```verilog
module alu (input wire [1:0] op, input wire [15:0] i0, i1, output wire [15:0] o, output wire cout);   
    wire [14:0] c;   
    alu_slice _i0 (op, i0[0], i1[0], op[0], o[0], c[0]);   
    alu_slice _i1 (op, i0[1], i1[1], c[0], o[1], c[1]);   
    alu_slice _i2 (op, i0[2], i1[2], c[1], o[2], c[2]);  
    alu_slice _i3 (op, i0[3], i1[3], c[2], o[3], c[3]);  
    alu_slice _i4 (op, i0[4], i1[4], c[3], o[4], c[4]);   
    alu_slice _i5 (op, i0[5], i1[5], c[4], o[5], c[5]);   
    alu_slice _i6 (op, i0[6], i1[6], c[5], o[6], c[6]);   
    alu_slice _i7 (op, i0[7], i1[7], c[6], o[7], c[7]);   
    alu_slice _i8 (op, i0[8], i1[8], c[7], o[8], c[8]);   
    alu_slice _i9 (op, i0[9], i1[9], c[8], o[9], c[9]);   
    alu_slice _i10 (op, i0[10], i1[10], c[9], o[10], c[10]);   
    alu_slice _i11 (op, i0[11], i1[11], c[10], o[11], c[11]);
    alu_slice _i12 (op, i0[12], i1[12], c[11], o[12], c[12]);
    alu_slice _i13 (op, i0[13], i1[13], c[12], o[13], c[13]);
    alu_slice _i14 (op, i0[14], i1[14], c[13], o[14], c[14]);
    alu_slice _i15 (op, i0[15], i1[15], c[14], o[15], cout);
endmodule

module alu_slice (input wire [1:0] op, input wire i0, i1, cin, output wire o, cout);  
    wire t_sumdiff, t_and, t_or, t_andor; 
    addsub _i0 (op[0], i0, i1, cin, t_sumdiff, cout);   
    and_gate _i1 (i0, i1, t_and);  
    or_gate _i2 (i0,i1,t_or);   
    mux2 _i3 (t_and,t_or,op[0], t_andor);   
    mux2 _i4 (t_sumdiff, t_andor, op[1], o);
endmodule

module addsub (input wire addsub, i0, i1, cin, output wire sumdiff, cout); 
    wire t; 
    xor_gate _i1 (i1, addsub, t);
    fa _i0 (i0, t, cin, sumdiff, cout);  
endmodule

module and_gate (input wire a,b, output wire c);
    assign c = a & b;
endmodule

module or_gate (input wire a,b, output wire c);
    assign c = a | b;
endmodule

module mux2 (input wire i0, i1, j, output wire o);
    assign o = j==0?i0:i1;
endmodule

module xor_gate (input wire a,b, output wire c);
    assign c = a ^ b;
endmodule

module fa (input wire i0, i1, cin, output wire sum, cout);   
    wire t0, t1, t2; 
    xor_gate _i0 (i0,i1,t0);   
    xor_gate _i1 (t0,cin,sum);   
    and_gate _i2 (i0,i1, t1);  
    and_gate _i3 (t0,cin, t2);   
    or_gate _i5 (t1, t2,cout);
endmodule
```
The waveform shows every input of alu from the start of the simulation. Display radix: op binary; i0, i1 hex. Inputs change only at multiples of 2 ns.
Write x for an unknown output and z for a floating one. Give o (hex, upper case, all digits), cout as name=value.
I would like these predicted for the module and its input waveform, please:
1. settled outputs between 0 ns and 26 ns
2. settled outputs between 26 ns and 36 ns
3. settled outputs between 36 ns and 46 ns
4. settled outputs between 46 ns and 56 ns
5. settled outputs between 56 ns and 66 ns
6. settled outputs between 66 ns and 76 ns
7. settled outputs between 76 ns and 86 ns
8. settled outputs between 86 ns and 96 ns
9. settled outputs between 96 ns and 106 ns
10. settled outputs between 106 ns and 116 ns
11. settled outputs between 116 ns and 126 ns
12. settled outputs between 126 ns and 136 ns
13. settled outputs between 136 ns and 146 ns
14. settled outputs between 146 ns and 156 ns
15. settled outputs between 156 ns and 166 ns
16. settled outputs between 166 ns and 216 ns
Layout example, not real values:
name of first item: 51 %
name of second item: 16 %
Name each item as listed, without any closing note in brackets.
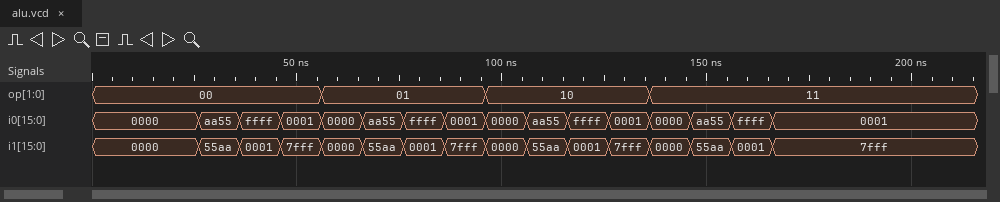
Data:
settled outputs between 0 ns and 26 ns: o=0000, cout=0
settled outputs between 26 ns and 36 ns: o=FFFF, cout=0
settled outputs between 36 ns and 46 ns: o=0000, cout=1
settled outputs between 46 ns and 56 ns: o=8000, cout=0
settled outputs between 56 ns and 66 ns: o=0000, cout=1
settled outputs between 66 ns and 76 ns: o=54AB, cout=1
settled outputs between 76 ns and 86 ns: o=FFFE, cout=1
settled outputs between 86 ns and 96 ns: o=8002, cout=0
settled outputs between 96 ns and 106 ns: o=0000, cout=0
settled outputs between 106 ns and 116 ns: o=0000, cout=0
settled outputs between 116 ns and 126 ns: o=0001, cout=1
settled outputs between 126 ns and 136 ns: o=0001, cout=0
settled outputs between 136 ns and 146 ns: o=0000, cout=1
settled outputs between 146 ns and 156 ns: o=FFFF, cout=1
settled outputs between 156 ns and 166 ns: o=FFFF, cout=1
settled outputs between 166 ns and 216 ns: o=7FFF, cout=0
